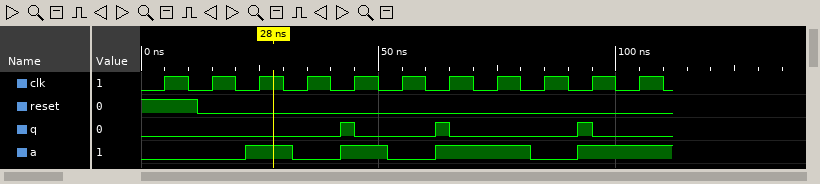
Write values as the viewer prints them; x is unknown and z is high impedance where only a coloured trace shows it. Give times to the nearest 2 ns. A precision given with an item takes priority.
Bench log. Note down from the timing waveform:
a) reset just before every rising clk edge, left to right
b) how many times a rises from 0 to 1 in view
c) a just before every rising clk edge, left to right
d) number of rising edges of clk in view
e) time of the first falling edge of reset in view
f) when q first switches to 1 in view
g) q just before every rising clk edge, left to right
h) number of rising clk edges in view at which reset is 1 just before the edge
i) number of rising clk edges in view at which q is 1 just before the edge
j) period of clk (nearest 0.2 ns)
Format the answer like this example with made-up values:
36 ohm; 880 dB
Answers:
1 0 0 0 0 0 0 0 0 0 0; 4; 0 0 1 0 1 0 1 1 0 1 1; 11; 12 ns; 42 ns; 0 0 0 0 1 0 1 0 0 1 0; 1; 3; 10 ns
